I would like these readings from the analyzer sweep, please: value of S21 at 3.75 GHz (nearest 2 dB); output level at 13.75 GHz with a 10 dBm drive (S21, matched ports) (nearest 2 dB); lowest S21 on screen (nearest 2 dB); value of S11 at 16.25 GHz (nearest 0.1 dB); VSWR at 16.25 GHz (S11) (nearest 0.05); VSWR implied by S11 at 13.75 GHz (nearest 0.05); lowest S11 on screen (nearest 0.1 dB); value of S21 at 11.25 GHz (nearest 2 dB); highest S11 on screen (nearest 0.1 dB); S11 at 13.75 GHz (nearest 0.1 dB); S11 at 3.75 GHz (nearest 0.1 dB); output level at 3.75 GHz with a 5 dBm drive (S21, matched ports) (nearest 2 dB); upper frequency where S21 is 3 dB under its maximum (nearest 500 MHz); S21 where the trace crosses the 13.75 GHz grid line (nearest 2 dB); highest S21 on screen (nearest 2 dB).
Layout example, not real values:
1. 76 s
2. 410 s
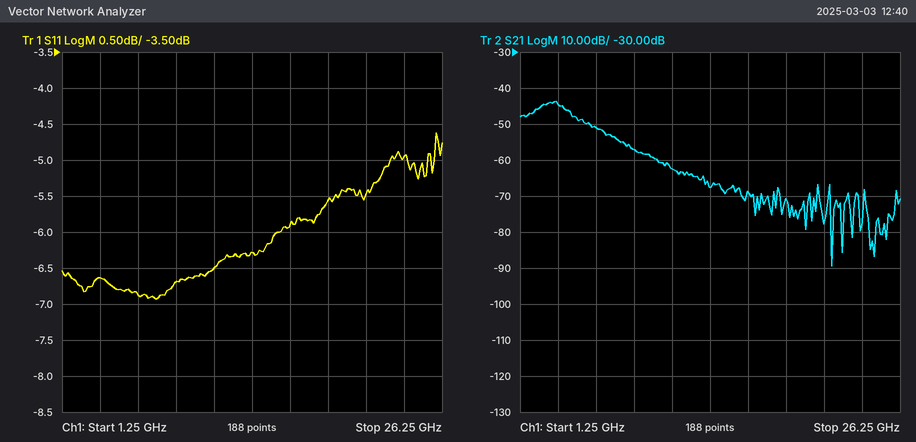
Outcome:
1. -44 dB
2. -58 dBm
3. -90 dB
4. -5.9 dB
5. 3.05
6. 2.90
7. -6.9 dB
8. -62 dB
9. -4.6 dB
10. -6.3 dB
11. -6.6 dB
12. -40 dBm
13. 4.5 GHz
14. -68 dB
15. -44 dB
